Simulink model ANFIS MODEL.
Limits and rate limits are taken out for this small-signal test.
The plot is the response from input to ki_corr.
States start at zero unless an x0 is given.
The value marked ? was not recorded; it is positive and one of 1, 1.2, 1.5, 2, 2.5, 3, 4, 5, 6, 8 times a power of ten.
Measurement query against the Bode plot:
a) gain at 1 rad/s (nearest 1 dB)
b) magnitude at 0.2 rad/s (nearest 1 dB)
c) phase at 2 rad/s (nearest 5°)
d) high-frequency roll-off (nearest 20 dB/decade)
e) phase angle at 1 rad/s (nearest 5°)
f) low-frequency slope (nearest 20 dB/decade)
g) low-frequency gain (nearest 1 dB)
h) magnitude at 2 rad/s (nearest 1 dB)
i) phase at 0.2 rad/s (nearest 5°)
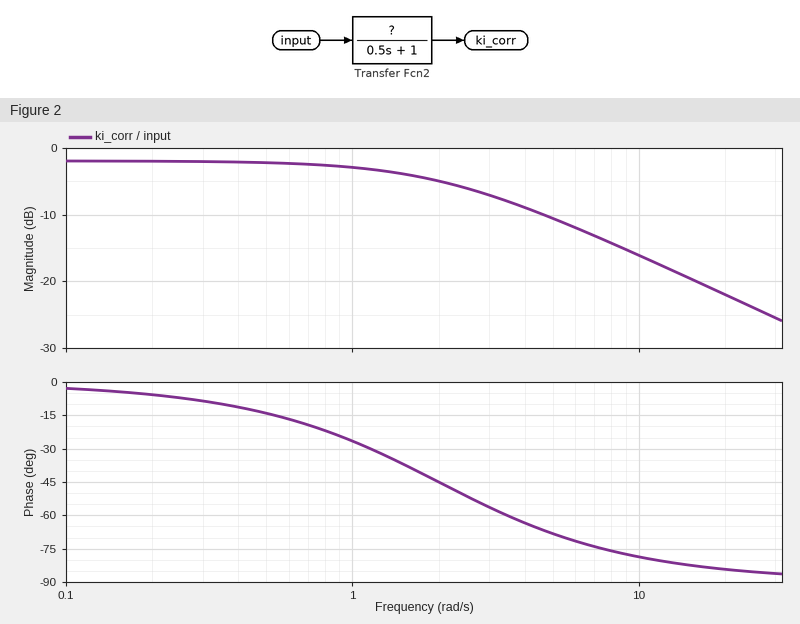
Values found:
-3 dB
-2 dB
-45°
-20 dB/decade
-25°
0 dB/decade
-2 dB
-5 dB
-5°
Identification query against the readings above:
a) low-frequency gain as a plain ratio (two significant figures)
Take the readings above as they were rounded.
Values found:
0.79
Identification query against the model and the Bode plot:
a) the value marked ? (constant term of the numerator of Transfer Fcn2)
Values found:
0.8
